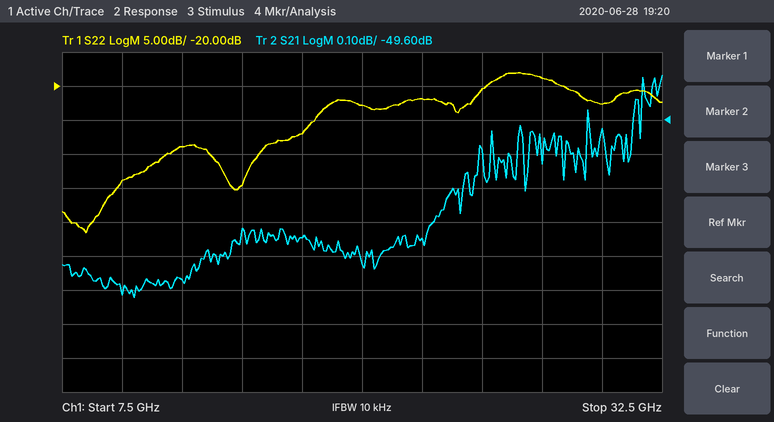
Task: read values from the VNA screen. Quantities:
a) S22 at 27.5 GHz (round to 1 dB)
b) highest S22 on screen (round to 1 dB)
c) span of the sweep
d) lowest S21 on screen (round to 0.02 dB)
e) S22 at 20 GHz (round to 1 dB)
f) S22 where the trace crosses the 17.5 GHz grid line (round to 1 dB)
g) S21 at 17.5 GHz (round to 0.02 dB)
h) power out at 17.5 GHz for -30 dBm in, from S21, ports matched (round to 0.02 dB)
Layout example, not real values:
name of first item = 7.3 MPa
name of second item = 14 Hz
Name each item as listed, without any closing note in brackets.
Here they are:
S22 at 27.5 GHz = -19 dB
highest S22 on screen = -18 dB
span of the sweep = 25 GHz
lowest S21 on screen = -50.12 dB
S22 at 20 GHz = -23 dB
S22 where the trace crosses the 17.5 GHz grid line = -27 dB
S21 at 17.5 GHz = -49.94 dB
power out at 17.5 GHz for -30 dBm in, from S21, ports matched = -79.94 dBm
